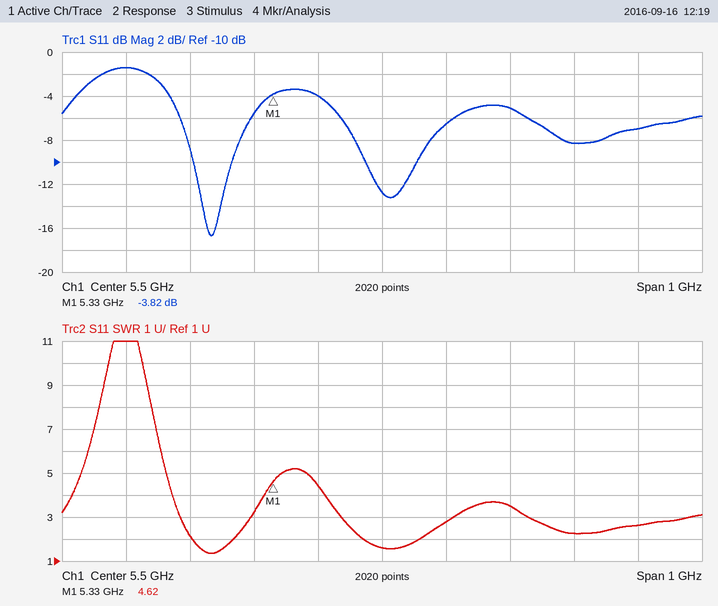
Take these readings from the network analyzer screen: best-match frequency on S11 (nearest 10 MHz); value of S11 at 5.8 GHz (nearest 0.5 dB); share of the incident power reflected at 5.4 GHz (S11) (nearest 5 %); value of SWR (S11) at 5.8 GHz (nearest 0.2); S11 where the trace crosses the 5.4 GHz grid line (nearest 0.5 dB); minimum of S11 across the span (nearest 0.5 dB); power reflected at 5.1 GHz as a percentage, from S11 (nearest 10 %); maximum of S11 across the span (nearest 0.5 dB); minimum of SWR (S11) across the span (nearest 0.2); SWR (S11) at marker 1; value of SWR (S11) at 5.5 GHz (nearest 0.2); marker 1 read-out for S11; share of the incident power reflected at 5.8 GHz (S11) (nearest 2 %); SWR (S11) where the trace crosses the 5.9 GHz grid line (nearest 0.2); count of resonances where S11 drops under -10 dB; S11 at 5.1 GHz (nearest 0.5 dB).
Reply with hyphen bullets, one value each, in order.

- 5.23 GHz
- -8.5 dB
- 40 %
- 2.2
- -4.0 dB
- -16.5 dB
- 70 %
- -1.5 dB
- 1.4
- 4.62
- 1.6
- -3.82 dB
- 14 %
- 2.6
- 2
- -1.5 dB
